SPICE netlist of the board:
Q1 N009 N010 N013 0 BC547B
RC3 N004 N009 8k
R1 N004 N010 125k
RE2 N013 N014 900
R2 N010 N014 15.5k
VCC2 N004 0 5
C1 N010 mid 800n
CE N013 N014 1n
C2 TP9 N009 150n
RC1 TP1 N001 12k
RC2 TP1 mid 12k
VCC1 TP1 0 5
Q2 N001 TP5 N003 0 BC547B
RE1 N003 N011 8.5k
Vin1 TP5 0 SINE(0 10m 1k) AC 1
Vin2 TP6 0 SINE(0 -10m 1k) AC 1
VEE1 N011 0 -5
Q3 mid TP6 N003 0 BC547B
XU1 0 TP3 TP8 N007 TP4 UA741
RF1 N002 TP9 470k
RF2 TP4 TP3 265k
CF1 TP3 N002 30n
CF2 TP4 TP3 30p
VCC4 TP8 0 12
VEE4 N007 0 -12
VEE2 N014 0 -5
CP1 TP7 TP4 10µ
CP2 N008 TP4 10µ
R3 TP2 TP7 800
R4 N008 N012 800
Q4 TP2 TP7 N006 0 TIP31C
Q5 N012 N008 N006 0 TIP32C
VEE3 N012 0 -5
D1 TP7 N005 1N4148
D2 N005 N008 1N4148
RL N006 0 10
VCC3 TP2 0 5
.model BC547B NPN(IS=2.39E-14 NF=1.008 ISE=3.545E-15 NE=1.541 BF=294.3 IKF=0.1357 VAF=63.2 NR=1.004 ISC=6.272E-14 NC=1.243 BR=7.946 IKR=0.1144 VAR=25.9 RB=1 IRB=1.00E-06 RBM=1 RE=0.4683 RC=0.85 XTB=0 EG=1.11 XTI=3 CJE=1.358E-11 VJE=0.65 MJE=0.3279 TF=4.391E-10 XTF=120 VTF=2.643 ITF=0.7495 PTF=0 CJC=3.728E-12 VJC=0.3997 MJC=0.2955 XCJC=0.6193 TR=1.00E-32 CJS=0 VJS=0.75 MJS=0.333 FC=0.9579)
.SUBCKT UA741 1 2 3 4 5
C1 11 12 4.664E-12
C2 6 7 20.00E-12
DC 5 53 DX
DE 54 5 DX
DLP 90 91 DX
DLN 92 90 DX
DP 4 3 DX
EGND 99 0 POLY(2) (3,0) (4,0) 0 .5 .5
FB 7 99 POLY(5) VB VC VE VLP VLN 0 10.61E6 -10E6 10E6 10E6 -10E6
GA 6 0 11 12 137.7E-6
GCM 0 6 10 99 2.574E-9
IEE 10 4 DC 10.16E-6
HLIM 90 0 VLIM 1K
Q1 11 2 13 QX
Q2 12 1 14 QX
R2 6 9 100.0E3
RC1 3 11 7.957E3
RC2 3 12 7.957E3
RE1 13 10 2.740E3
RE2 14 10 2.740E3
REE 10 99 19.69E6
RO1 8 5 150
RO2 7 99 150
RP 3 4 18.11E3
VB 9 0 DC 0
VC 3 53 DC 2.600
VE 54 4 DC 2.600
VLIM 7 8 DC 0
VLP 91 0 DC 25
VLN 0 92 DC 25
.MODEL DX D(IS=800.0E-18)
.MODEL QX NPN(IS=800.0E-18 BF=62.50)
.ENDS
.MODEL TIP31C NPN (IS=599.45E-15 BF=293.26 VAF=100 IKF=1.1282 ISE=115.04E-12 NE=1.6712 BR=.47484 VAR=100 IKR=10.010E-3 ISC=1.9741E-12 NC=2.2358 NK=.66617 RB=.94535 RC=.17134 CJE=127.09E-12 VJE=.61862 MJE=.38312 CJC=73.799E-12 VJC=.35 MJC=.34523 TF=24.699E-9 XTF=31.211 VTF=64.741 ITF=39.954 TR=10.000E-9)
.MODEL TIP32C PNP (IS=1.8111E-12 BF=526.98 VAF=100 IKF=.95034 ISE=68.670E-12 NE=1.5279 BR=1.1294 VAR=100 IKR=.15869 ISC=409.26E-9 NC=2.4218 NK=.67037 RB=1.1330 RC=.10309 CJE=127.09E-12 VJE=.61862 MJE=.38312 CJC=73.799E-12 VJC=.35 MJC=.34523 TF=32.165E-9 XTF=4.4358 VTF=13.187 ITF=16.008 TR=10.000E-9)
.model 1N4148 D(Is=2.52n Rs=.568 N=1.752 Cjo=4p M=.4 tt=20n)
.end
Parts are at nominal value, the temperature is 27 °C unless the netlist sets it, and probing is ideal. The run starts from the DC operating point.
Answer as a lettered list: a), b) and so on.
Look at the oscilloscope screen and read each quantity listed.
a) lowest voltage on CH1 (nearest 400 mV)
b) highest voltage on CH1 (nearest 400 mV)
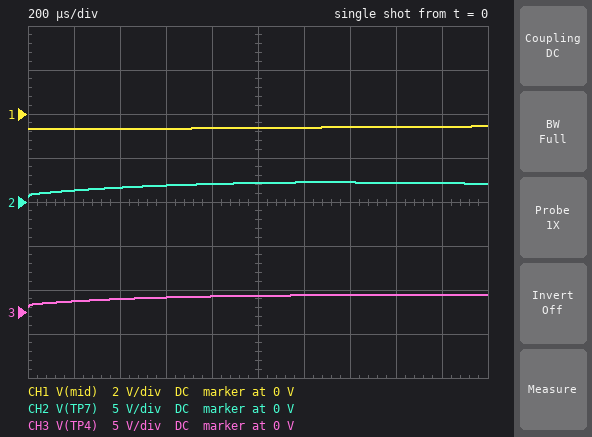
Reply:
a) -800 mV
b) -400 mV
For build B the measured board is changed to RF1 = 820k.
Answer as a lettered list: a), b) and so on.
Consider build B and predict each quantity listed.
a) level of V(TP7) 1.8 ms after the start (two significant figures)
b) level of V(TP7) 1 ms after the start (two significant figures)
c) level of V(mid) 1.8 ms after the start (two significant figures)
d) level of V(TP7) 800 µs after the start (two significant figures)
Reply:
a) 1.6 V
b) 1.5 V
c) -590 mV
d) 1.4 V
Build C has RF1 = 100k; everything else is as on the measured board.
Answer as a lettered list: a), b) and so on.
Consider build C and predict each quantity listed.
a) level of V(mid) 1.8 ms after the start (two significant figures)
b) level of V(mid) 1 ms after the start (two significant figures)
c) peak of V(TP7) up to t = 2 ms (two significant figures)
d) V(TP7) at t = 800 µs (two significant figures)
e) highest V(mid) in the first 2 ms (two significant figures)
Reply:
a) 1.4 V
b) 1.9 V
c) 5.5 V
d) -4.4 V
e) 2.5 V
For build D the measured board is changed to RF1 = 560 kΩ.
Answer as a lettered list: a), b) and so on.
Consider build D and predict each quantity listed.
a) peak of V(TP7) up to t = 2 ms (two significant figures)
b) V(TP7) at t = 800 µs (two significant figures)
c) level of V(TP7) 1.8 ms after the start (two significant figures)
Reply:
a) 2.0 V
b) 1.8 V
c) 1.9 V
